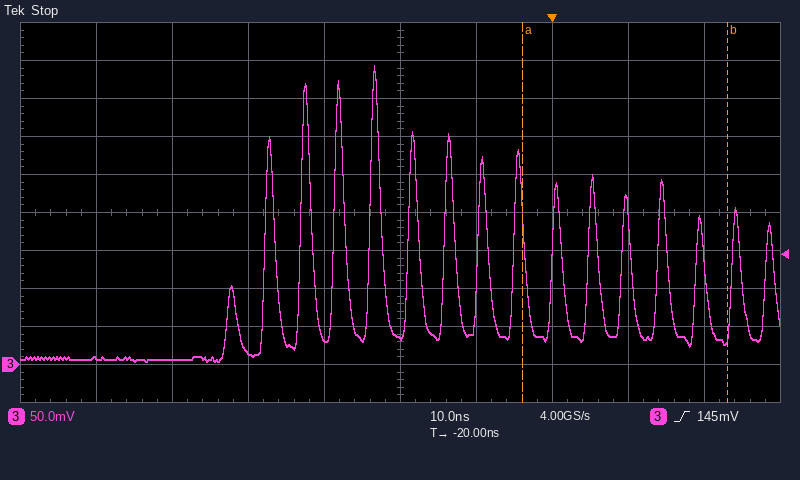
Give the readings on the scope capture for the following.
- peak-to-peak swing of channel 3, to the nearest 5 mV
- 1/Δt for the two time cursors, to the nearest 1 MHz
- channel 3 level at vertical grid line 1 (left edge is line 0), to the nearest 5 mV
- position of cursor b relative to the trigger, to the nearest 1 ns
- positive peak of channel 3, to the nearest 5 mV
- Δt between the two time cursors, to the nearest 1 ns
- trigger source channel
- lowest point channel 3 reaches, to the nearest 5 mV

390 mV
37 MHz
10 mV
+23 ns
395 mV
27 ns
channel 3
5 mV
